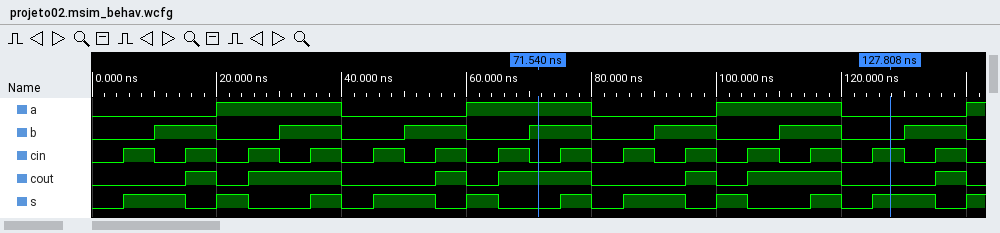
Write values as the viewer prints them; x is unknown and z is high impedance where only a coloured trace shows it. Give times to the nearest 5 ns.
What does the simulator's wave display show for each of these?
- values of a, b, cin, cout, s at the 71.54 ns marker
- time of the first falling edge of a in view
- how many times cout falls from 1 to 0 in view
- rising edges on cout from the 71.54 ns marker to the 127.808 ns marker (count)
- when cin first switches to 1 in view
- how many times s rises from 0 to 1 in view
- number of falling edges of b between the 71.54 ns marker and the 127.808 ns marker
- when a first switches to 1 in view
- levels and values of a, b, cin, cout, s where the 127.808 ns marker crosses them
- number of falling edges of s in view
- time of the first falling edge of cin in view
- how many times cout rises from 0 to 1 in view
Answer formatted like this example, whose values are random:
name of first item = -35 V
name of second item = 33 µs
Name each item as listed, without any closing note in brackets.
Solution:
values of a, b, cin, cout, s at the 71.54 ns marker = a=1, b=1, cin=0, cout=1, s=0
time of the first falling edge of a in view = 40 ns
how many times cout falls from 1 to 0 in view = 7
rising edges on cout from the 71.54 ns marker to the 127.808 ns marker = 2
when cin first switches to 1 in view = 5 ns
how many times s rises from 0 to 1 in view = 11
number of falling edges of b between the 71.54 ns marker and the 127.808 ns marker = 3
when a first switches to 1 in view = 20 ns
levels and values of a, b, cin, cout, s where the 127.808 ns marker crosses them = a=0, b=0, cin=1, cout=0, s=1
number of falling edges of s in view = 10
time of the first falling edge of cin in view = 10 ns
how many times cout rises from 0 to 1 in view = 7
